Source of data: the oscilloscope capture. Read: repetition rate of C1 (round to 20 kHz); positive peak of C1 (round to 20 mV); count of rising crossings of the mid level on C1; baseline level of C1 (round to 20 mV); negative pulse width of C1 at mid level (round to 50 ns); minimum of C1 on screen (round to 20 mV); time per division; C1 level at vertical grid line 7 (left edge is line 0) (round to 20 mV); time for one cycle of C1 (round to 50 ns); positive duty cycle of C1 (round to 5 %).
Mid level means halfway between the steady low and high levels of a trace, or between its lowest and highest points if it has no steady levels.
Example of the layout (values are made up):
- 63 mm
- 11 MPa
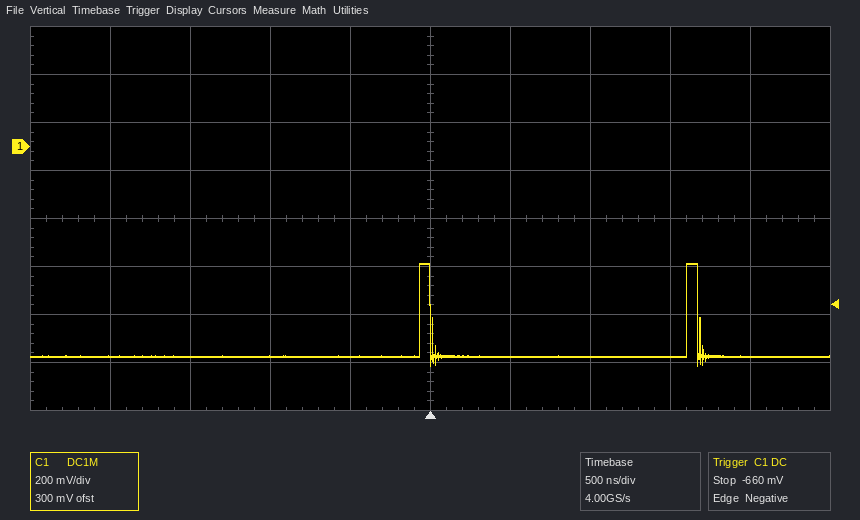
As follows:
- 600 kHz
- -480 mV
- 2
- -880 mV
- 1.60 µs
- -920 mV
- 500 ns
- -880 mV
- 1.65 µs
- 5 %
